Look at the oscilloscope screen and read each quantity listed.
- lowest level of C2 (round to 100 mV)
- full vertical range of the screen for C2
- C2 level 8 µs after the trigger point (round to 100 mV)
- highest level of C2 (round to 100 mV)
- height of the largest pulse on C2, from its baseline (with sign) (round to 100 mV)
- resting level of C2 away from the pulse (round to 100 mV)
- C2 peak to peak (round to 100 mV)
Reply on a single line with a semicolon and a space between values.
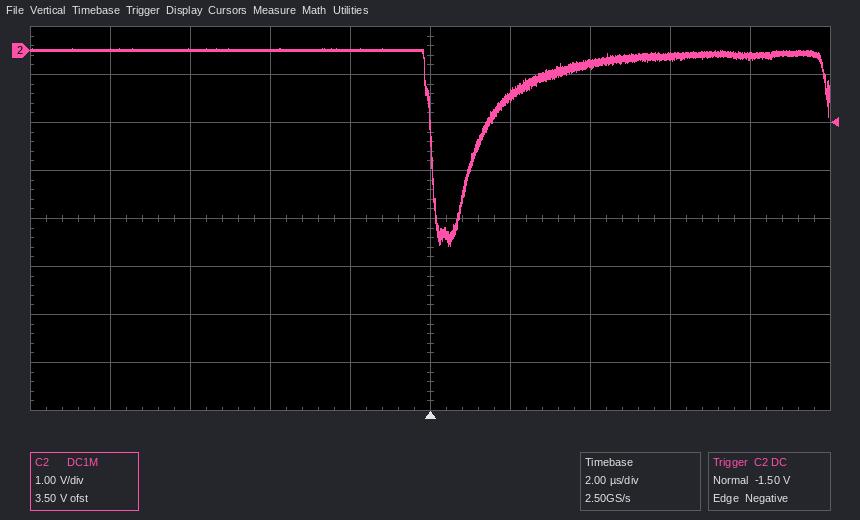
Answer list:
-4.1 V; 8 V; -100 mV; 0.0 V; -4.1 V; 0.0 V; 4.1 V
